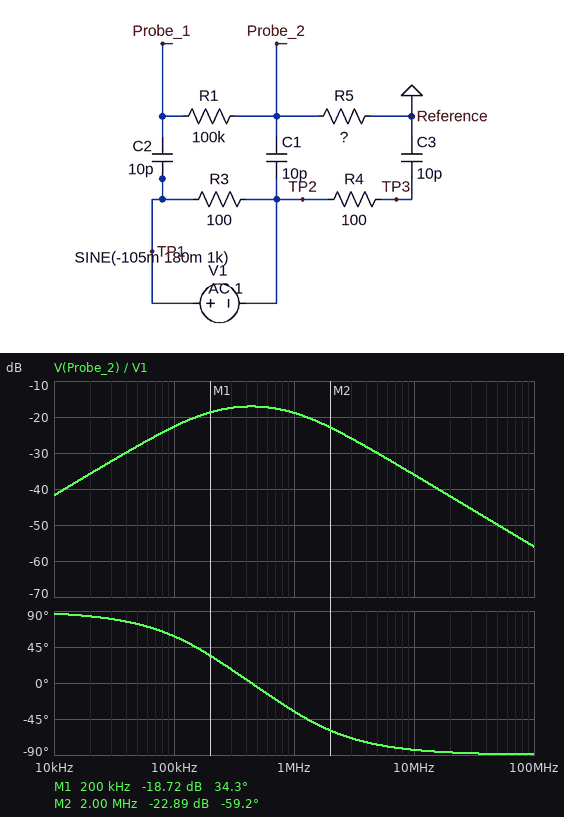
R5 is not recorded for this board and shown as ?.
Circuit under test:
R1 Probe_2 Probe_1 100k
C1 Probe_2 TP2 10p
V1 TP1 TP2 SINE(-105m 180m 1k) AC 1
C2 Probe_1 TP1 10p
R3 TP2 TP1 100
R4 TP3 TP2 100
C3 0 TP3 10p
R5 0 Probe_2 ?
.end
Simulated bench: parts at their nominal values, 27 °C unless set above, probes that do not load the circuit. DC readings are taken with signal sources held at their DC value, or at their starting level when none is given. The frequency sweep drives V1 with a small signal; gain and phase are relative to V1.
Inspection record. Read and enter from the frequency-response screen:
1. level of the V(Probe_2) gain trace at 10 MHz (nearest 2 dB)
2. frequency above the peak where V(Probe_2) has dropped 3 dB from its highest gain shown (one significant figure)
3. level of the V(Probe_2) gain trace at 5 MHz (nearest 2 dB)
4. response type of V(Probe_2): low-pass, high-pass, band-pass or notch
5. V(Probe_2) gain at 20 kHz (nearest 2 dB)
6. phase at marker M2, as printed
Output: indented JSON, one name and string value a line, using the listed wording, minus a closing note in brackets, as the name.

{
  "level of the V(Probe_2) gain trace at 10 MHz": "-36 dB",
  "frequency above the peak where V(Probe_2) has dropped 3 dB from its highest gain shown": "1 MHz",
  "level of the V(Probe_2) gain trace at 5 MHz": "-30 dB",
  "response type of V(Probe_2): low-pass, high-pass, band-pass or notch": "band-pass",
  "V(Probe_2) gain at 20 kHz": "-36 dB",
  "phase at marker M2, as printed": "-59.2 deg"
}
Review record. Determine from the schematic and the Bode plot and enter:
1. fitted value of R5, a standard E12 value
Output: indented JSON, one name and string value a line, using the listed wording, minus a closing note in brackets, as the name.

{
  "fitted value of R5, a standard E12 value": "39 kΩ"
}
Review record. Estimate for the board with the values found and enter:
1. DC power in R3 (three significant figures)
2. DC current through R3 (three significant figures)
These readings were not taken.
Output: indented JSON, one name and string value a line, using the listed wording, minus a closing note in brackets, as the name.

{
  "DC power in R3": "110 µW",
  "DC current through R3": "1.05 mA"
}
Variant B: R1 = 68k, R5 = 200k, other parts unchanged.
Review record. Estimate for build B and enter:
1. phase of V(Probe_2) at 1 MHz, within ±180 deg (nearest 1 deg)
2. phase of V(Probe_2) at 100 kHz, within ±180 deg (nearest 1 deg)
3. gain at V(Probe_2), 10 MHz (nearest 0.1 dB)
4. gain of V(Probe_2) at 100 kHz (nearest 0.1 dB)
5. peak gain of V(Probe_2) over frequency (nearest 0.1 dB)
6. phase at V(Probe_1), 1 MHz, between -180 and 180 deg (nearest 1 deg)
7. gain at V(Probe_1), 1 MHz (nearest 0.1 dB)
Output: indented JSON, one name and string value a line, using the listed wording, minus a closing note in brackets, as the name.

{
  "phase of V(Probe_2) at 1 MHz, within ±180 deg": "-56 deg",
  "phase of V(Probe_2) at 100 kHz, within ±180 deg": "36 deg",
  "gain at V(Probe_2), 10 MHz": "-32.6 dB",
  "gain of V(Probe_2) at 100 kHz": "-10.4 dB",
  "peak gain of V(Probe_2) over frequency": "-8.6 dB",
  "phase at V(Probe_1), 1 MHz, between -180 and 180 deg": "12 deg",
  "gain at V(Probe_1), 1 MHz": "-0.5 dB"
}
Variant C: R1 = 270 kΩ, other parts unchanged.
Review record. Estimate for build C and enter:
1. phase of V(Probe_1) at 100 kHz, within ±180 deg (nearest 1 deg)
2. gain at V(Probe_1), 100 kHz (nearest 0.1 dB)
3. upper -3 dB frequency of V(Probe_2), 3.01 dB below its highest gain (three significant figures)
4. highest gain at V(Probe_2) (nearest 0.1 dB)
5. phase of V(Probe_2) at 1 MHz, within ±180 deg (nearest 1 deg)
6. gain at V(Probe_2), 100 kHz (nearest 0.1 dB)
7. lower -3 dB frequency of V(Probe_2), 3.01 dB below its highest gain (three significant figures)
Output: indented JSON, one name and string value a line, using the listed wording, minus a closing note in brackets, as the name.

{
  "phase of V(Probe_1) at 100 kHz, within ±180 deg": "40 deg",
  "gain at V(Probe_1), 100 kHz": "-2.1 dB",
  "upper -3 dB frequency of V(Probe_2), 3.01 dB below its highest gain": "1.00 MHz",
  "highest gain at V(Probe_2)": "-24.0 dB",
  "phase of V(Probe_2) at 1 MHz, within ±180 deg": "-45 deg",
  "gain at V(Probe_2), 100 kHz": "-25.6 dB",
  "lower -3 dB frequency of V(Probe_2), 3.01 dB below its highest gain": "71.7 kHz"
}
